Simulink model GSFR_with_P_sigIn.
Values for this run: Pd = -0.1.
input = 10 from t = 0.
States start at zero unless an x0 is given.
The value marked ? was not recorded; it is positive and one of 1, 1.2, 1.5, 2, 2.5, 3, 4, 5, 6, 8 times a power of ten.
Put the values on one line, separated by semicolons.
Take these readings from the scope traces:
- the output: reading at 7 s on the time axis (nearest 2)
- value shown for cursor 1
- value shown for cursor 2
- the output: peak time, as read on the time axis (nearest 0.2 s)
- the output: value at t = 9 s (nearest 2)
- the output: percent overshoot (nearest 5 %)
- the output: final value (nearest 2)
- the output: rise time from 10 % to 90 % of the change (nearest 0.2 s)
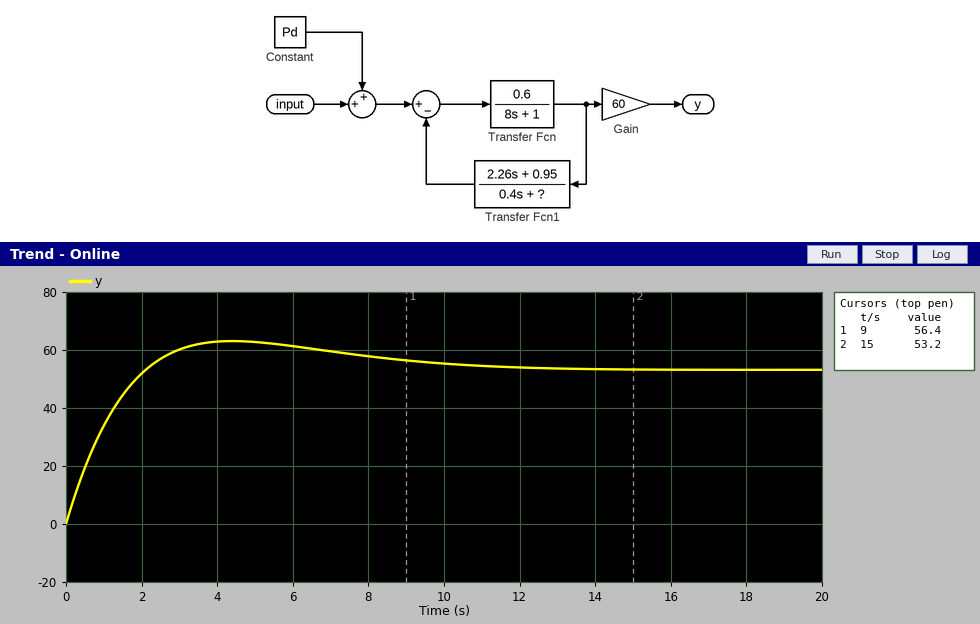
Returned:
60; 56.4; 53.2; 4.4 s; 56; 20 %; 54; 1.6 s
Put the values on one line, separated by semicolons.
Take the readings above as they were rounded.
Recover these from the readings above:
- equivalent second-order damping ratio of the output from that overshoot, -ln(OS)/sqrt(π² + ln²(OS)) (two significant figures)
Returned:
0.46
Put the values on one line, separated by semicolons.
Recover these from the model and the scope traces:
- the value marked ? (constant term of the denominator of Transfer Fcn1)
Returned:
0.1
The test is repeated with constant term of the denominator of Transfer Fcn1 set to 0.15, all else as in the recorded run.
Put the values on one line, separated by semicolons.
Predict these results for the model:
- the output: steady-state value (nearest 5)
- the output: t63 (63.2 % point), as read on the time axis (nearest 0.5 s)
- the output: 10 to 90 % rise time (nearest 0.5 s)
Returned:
75; 1.5 s; 3.0 s
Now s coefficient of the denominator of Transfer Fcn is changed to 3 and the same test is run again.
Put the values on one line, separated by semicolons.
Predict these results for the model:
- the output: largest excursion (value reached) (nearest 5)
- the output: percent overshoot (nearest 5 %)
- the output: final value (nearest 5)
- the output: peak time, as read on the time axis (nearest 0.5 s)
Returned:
70; 30 %; 55; 2.0 s
